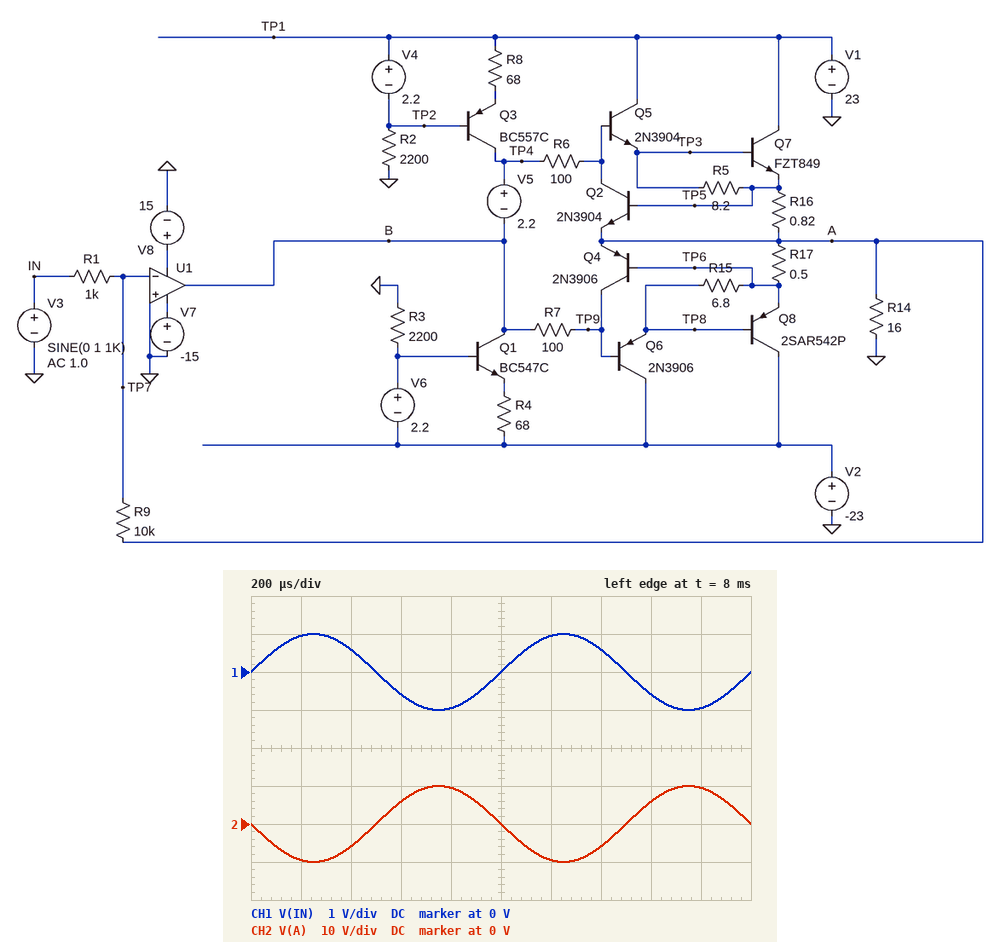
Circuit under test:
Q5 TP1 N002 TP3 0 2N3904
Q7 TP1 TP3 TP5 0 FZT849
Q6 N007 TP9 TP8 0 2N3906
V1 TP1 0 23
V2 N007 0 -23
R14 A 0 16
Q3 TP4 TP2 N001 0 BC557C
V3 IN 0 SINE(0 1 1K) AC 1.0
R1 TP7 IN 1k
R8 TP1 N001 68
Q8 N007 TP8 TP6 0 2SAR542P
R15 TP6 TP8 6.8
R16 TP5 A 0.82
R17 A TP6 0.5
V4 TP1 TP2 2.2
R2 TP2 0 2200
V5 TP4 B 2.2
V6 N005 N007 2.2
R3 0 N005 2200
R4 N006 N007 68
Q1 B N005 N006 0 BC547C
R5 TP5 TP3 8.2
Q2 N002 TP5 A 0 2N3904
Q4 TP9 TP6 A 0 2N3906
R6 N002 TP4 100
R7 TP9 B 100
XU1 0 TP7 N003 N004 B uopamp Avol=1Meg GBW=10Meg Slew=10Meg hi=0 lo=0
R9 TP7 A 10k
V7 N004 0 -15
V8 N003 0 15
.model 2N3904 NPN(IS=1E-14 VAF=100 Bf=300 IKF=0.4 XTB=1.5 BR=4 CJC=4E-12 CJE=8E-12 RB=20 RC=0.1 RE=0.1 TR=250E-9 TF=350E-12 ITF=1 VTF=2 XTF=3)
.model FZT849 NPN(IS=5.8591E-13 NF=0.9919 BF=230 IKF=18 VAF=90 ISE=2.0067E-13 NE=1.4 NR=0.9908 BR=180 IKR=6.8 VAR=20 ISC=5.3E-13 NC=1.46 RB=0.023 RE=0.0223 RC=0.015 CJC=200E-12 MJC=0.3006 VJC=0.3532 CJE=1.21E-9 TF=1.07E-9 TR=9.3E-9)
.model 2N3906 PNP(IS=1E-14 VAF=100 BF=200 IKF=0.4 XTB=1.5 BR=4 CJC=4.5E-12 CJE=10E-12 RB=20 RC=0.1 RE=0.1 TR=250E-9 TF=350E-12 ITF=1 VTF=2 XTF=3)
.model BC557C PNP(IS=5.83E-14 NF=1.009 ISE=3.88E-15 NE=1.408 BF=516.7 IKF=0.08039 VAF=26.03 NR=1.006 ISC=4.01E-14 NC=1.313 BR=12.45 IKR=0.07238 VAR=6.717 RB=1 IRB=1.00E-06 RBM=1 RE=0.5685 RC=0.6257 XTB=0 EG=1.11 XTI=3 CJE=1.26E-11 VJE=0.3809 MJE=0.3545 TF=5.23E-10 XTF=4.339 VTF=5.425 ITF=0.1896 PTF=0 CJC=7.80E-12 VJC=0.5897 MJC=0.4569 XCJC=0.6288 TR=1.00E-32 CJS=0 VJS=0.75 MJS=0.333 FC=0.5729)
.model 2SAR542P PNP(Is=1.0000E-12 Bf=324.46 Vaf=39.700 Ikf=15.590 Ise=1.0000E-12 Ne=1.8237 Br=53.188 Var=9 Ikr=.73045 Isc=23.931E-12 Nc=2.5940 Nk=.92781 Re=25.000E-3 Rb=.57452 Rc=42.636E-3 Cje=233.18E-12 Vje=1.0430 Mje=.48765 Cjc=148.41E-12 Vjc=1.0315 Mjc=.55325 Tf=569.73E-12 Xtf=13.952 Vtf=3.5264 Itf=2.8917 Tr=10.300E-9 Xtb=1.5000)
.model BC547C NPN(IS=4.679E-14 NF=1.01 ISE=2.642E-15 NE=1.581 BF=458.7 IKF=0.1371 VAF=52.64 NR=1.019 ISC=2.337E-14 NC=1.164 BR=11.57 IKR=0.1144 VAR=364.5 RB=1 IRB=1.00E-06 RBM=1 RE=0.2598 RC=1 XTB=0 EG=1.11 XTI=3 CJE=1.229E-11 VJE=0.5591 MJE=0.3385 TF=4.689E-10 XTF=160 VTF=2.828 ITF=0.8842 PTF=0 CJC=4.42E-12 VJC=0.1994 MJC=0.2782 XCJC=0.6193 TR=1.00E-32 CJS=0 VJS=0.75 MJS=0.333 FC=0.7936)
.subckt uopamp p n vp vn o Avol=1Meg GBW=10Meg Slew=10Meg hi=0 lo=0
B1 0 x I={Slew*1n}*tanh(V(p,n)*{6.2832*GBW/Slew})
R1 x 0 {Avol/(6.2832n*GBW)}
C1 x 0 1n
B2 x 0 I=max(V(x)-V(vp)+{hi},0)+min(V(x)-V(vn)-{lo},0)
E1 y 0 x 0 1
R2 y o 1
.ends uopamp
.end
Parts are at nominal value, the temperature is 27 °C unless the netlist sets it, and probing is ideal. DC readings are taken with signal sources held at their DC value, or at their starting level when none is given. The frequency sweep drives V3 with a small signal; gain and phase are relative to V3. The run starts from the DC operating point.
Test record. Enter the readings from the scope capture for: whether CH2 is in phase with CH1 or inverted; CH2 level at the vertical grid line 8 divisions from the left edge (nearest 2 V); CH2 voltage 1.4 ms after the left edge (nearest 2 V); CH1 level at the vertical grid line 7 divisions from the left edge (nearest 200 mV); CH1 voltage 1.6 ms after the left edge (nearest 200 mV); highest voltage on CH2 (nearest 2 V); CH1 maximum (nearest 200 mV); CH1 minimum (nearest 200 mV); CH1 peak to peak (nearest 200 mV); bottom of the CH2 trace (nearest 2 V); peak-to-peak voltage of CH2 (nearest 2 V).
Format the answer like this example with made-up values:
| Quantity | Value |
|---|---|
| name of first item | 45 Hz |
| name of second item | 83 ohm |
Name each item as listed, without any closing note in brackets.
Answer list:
| Quantity | Value |
|---|---|
| whether CH2 is in phase with CH1 or inverted | inverted |
| CH2 level at the vertical grid line 8 divisions from the left edge | 6 V |
| CH2 voltage 1.4 ms after the left edge | -6 V |
| CH1 level at the vertical grid line 7 divisions from the left edge | 600 mV |
| CH1 voltage 1.6 ms after the left edge | -600 mV |
| highest voltage on CH2 | 10 V |
| CH1 maximum | 1.0 V |
| CH1 minimum | -1.0 V |
| CH1 peak to peak | 2.0 V |
| bottom of the CH2 trace | -10 V |
| peak-to-peak voltage of CH2 | 20 V |
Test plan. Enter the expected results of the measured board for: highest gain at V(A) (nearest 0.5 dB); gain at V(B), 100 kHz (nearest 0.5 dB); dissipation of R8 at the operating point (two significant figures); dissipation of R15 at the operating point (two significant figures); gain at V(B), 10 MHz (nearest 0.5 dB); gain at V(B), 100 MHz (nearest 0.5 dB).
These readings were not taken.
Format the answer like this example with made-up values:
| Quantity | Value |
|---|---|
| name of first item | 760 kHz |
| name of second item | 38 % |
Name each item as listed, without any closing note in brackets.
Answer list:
| Quantity | Value |
|---|---|
| highest gain at V(A) | 20.0 dB |
| gain at V(B), 100 kHz | 22.0 dB |
| dissipation of R8 at the operating point | 33 mW |
| dissipation of R15 at the operating point | 11 mW |
| gain at V(B), 10 MHz | -1.0 dB |
| gain at V(B), 100 MHz | -21.0 dB |
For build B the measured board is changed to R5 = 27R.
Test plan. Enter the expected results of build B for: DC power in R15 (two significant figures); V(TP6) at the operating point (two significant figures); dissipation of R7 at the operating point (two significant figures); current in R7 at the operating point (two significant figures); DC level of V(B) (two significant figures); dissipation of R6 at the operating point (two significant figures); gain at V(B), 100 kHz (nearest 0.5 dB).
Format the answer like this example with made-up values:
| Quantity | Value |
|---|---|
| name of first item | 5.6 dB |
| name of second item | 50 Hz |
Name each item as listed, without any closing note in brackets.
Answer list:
| Quantity | Value |
|---|---|
| DC power in R15 | 3.1 mW |
| V(TP6) at the operating point | -11 mV |
| dissipation of R7 at the operating point | 830 nW |
| current in R7 at the operating point | 91 µA |
| DC level of V(B) | -900 mV |
| dissipation of R6 at the operating point | 330 nW |
| gain at V(B), 100 kHz | 22.5 dB |
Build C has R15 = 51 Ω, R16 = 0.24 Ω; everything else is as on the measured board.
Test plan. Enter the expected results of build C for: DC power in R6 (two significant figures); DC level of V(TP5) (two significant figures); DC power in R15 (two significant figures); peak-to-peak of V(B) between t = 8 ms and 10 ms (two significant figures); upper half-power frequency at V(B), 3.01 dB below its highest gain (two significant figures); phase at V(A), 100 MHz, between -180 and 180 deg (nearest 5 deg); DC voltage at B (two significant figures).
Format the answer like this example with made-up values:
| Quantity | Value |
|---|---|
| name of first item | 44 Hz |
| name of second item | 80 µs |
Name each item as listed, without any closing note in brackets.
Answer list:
| Quantity | Value |
|---|---|
| DC power in R6 | 280 nW |
| DC level of V(TP5) | 4.5 mV |
| DC power in R15 | 6.5 mW |
| peak-to-peak of V(B) between t = 8 ms and 10 ms | 21 V |
| upper half-power frequency at V(B), 3.01 dB below its highest gain | 770 kHz |
| phase at V(A), 100 MHz, between -180 and 180 deg | 15 deg |
| DC voltage at B | -1.3 V |
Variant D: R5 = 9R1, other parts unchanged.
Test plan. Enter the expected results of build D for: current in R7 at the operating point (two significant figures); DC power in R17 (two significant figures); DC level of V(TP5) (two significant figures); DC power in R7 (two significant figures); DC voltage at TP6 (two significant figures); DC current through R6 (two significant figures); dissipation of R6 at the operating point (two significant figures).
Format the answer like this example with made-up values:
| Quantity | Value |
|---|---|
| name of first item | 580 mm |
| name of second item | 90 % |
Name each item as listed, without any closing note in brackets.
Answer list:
| Quantity | Value |
|---|---|
| current in R7 at the operating point | 170 µA |
| DC power in R17 | 750 µW |
| DC level of V(TP5) | 32 mV |
| DC power in R7 | 2.9 µW |
| DC voltage at TP6 | -19 mV |
| DC current through R6 | 110 µA |
| dissipation of R6 at the operating point | 1.3 µW |
